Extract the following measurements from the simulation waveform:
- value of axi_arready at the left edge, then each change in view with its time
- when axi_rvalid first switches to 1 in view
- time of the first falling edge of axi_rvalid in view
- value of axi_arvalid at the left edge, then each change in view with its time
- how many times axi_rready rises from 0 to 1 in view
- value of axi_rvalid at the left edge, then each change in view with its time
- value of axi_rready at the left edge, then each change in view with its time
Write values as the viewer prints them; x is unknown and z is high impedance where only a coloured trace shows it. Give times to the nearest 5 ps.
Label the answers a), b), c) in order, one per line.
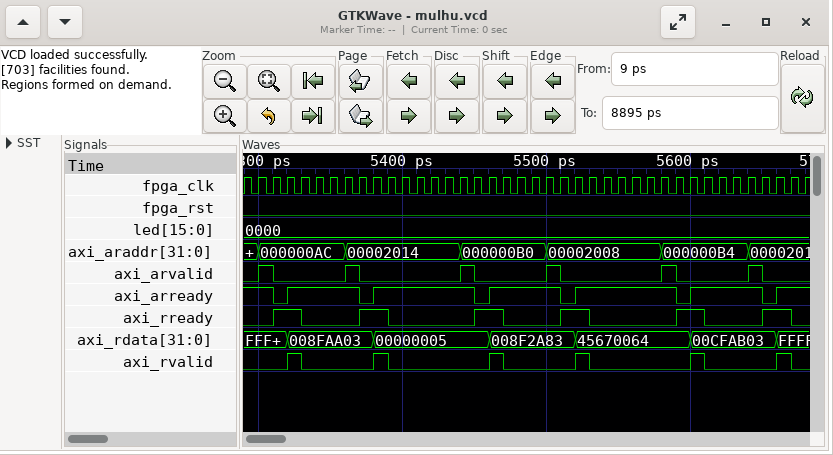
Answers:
a) 1, 0 at 5310 ps, 1 at 5320 ps, 0 at 5370 ps, 1 at 5380 ps, 0 at 5450 ps, 1 at 5460 ps, 0 at 5510 ps, 1 at 5520 ps, 0 at 5590 ps, 1 at 5600 ps, 0 at 5650 ps, 1 at 5660 ps
b) 5320 ps
c) 5330 ps
d) 0, 1 at 5300 ps, 0 at 5310 ps, 1 at 5360 ps, 0 at 5370 ps, 1 at 5440 ps, 0 at 5450 ps, 1 at 5500 ps, 0 at 5510 ps, 1 at 5580 ps, 0 at 5590 ps, 1 at 5640 ps, 0 at 5650 ps
e) 6
f) 0, 1 at 5320 ps, 0 at 5330 ps, 1 at 5380 ps, 0 at 5390 ps, 1 at 5460 ps, 0 at 5470 ps, 1 at 5520 ps, 0 at 5530 ps, 1 at 5600 ps, 0 at 5610 ps, 1 at 5660 ps, 0 at 5670 ps
g) 0, 1 at 5310 ps, 0 at 5330 ps, 1 at 5370 ps, 0 at 5390 ps, 1 at 5450 ps, 0 at 5470 ps, 1 at 5510 ps, 0 at 5530 ps, 1 at 5590 ps, 0 at 5610 ps, 1 at 5650 ps, 0 at 5670 ps
